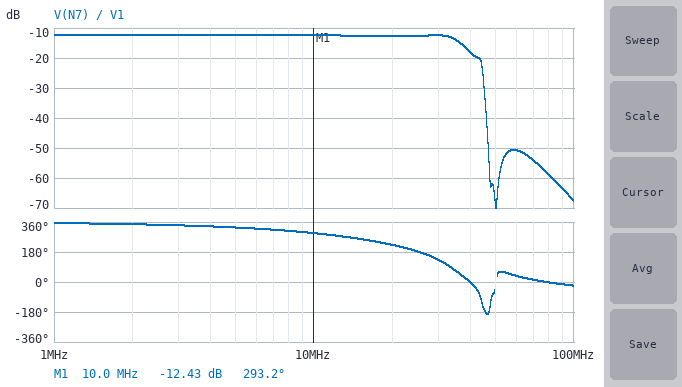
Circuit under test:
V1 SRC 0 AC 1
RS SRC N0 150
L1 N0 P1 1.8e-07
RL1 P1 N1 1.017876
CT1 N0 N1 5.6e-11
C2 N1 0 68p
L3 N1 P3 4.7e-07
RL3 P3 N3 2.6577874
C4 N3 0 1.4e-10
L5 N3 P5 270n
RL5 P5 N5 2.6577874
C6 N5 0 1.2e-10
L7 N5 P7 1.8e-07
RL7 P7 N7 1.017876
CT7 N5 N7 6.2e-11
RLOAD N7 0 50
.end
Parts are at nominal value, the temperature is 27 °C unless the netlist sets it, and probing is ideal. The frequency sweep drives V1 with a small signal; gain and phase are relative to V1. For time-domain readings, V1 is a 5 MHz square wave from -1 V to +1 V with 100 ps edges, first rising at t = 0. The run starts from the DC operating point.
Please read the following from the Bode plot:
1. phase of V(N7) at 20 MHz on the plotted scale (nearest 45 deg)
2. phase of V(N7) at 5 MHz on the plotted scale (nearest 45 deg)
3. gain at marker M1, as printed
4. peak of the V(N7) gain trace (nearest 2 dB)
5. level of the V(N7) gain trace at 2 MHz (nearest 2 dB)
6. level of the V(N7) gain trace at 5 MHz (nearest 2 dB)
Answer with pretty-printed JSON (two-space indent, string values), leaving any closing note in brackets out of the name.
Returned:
{
  "phase of V(N7) at 20 MHz on the plotted scale": "225 deg",
  "phase of V(N7) at 5 MHz on the plotted scale": "315 deg",
  "gain at marker M1, as printed": "-12.43 dB",
  "peak of the V(N7) gain trace": "-12 dB",
  "level of the V(N7) gain trace at 2 MHz": "-12 dB",
  "level of the V(N7) gain trace at 5 MHz": "-12 dB"
}
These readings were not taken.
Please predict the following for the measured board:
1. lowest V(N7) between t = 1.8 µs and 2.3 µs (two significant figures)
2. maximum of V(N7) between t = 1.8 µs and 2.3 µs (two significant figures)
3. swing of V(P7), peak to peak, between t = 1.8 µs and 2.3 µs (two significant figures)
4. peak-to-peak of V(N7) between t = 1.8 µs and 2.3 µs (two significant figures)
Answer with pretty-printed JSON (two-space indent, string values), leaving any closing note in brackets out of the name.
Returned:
{
  "lowest V(N7) between t = 1.8 µs and 2.3 µs": "-320 mV",
  "maximum of V(N7) between t = 1.8 µs and 2.3 µs": "320 mV",
  "swing of V(P7), peak to peak, between t = 1.8 µs and 2.3 µs": "650 mV",
  "peak-to-peak of V(N7) between t = 1.8 µs and 2.3 µs": "630 mV"
}
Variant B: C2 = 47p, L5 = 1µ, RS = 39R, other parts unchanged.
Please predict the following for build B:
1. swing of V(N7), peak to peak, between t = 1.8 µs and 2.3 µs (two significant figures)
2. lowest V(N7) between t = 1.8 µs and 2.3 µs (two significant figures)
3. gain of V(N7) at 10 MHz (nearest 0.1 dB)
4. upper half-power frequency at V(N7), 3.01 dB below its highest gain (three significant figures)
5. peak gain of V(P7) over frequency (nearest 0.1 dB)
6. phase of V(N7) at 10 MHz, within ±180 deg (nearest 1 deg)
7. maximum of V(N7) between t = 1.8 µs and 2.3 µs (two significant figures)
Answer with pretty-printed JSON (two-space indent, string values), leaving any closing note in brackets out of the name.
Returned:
{
  "swing of V(N7), peak to peak, between t = 1.8 µs and 2.3 µs": "1.2 V",
  "lowest V(N7) between t = 1.8 µs and 2.3 µs": "-610 mV",
  "gain of V(N7) at 10 MHz": "-6.7 dB",
  "upper half-power frequency at V(N7), 3.01 dB below its highest gain": "24.7 MHz",
  "peak gain of V(P7) over frequency": "-5.5 dB",
  "phase of V(N7) at 10 MHz, within ±180 deg": "-87 deg",
  "maximum of V(N7) between t = 1.8 µs and 2.3 µs": "610 mV"
}
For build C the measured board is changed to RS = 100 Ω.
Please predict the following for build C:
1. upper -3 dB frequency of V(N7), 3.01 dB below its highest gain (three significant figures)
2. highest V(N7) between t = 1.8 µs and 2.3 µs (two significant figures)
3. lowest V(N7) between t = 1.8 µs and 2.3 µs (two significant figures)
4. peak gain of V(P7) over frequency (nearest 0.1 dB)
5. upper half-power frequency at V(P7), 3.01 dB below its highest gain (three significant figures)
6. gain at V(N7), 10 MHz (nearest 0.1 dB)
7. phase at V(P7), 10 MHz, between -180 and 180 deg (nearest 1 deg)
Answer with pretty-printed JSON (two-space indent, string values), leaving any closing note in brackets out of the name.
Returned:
{
  "upper -3 dB frequency of V(N7), 3.01 dB below its highest gain": "37.3 MHz",
  "highest V(N7) between t = 1.8 µs and 2.3 µs": "410 mV",
  "lowest V(N7) between t = 1.8 µs and 2.3 µs": "-410 mV",
  "peak gain of V(P7) over frequency": "-9.8 dB",
  "upper half-power frequency at V(P7), 3.01 dB below its highest gain": "37.7 MHz",
  "gain at V(N7), 10 MHz": "-10.0 dB",
  "phase at V(P7), 10 MHz, between -180 and 180 deg": "-68 deg"
}
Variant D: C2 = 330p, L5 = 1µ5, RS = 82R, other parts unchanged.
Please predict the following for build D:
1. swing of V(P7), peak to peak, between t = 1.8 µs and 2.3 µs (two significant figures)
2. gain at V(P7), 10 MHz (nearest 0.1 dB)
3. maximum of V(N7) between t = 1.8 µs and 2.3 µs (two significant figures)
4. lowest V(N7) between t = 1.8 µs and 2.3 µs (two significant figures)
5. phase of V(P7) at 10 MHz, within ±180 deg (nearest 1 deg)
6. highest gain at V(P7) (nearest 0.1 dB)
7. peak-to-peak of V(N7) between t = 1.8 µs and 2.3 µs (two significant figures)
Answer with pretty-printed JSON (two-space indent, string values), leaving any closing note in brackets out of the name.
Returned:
{
  "swing of V(P7), peak to peak, between t = 1.8 µs and 2.3 µs": "940 mV",
  "gain at V(P7), 10 MHz": "-12.5 dB",
  "maximum of V(N7) between t = 1.8 µs and 2.3 µs": "460 mV",
  "lowest V(N7) between t = 1.8 µs and 2.3 µs": "-460 mV",
  "phase of V(P7) at 10 MHz, within ±180 deg": "-145 deg",
  "highest gain at V(P7)": "-8.5 dB",
  "peak-to-peak of V(N7) between t = 1.8 µs and 2.3 µs": "920 mV"
}
